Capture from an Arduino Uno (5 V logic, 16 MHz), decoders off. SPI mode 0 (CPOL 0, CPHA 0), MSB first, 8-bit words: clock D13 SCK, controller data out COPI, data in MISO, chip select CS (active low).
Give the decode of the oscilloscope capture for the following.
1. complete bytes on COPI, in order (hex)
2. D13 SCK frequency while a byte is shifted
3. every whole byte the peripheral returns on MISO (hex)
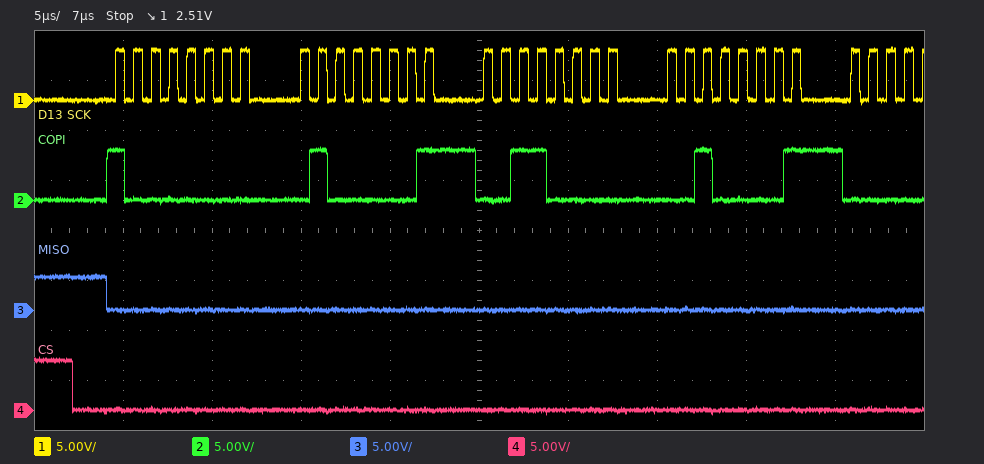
80 41 30 21
1 MHz
00 00 00 00
